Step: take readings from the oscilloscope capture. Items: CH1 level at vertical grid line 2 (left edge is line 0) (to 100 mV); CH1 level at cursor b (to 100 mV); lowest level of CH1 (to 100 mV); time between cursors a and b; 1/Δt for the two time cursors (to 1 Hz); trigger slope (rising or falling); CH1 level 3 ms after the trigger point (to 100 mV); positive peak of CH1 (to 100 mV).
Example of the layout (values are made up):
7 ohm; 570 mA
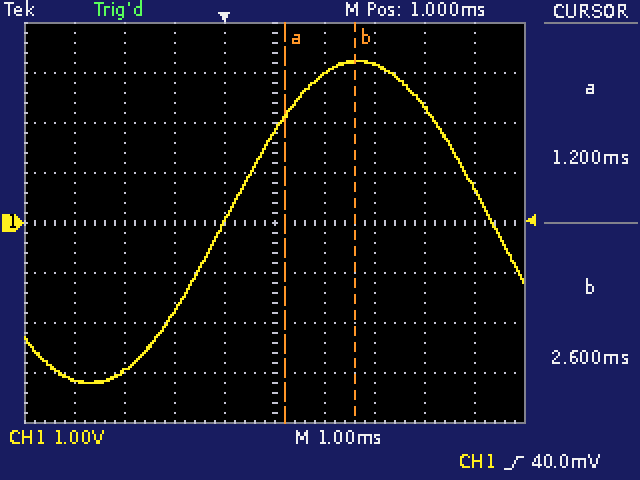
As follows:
-3.0 V; 3.2 V; -3.2 V; 1.4 ms; 714 Hz; rising; 3.2 V; 3.2 V
